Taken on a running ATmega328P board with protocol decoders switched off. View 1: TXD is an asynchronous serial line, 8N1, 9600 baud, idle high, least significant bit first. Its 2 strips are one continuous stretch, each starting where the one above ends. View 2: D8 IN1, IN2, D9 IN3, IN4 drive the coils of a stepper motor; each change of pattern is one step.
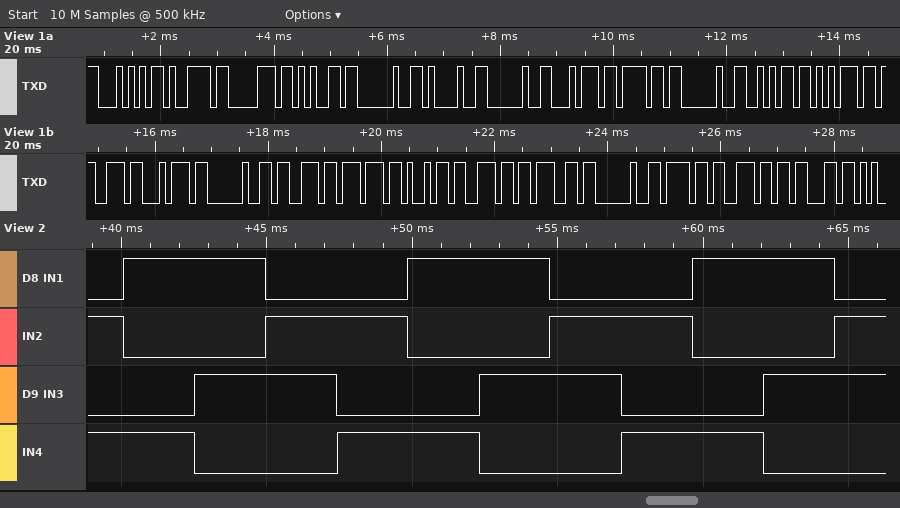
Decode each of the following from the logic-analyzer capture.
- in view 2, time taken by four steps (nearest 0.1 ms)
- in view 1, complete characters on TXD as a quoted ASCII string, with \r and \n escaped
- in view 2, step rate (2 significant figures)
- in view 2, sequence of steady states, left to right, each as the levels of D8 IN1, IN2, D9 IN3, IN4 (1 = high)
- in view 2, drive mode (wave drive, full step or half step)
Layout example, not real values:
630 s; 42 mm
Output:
9.8 ms; "Type ! to just swing onc"; 410 steps/s; 0101 1001 1010 0110 0101 1001 1010 0110 0101 1001 1010 0110; full step
